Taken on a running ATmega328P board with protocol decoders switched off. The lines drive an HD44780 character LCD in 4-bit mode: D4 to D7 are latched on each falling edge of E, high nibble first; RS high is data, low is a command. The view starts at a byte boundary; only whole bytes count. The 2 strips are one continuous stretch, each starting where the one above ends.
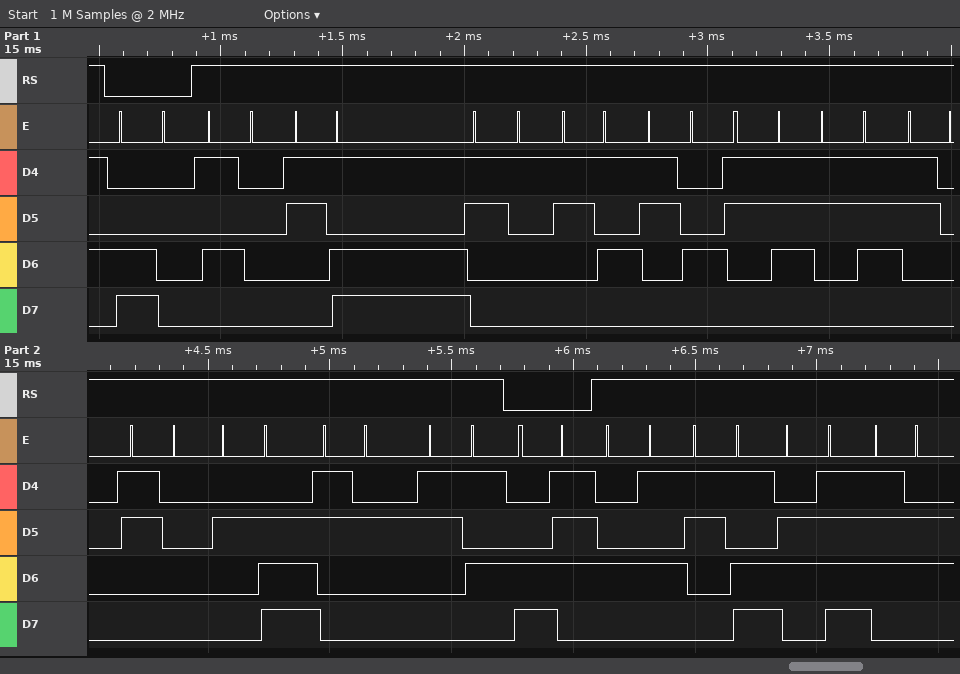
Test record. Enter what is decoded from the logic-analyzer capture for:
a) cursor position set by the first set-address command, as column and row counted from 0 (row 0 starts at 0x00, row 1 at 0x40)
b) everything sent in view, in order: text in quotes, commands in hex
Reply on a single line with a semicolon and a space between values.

column 0, row 1; 0xC0 "P=1547700.25" 0xC7 "E=ov"
